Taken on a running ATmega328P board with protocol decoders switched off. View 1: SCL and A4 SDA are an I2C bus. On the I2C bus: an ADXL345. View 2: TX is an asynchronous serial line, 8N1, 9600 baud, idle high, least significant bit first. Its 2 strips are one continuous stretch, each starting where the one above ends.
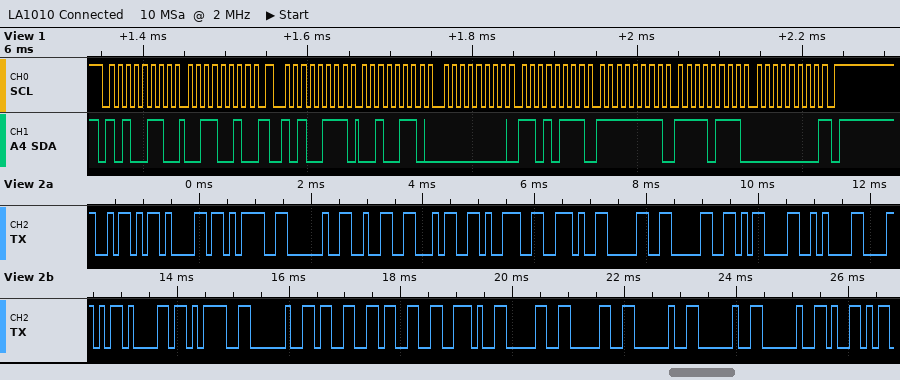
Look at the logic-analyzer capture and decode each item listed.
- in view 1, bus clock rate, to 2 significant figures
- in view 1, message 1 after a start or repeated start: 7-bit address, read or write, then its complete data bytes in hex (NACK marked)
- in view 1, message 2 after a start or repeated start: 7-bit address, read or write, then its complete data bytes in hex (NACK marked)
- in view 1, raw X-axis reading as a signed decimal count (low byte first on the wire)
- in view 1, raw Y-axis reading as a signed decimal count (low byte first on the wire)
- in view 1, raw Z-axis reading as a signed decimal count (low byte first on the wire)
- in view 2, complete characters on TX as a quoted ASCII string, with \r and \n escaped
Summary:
100 kHz
0x53 write: 32
0x53 read: 26 00 D7 FF F7 00 NACK
38
-41
247
"Za= 249.00\r\nXa= 33.00   Y"
